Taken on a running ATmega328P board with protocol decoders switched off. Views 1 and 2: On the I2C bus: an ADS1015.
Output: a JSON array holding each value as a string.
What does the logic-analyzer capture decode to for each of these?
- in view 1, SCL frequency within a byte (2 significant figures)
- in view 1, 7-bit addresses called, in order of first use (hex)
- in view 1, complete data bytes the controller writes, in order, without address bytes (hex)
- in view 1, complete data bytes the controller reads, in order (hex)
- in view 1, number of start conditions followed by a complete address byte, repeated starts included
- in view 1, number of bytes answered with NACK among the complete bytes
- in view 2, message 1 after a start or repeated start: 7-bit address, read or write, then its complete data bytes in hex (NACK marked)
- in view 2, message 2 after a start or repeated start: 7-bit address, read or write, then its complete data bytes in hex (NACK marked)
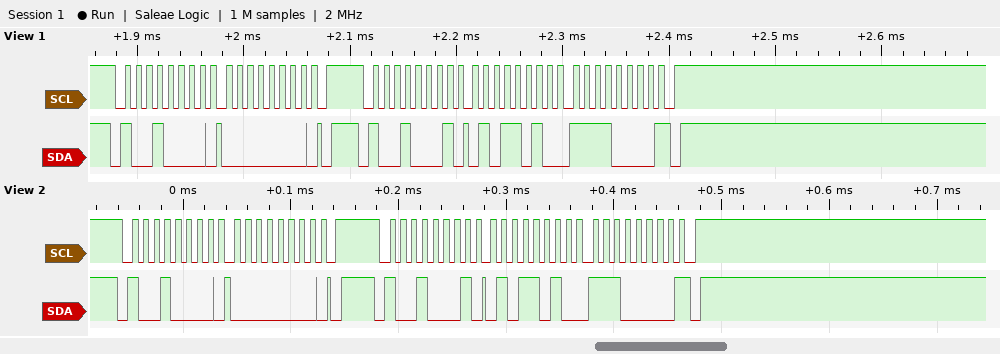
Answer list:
["100 kHz", "0x48", "00", "5A F0", "2", "1", "0x48 write: 00", "0x48 read: 5A E0 NACK"]
